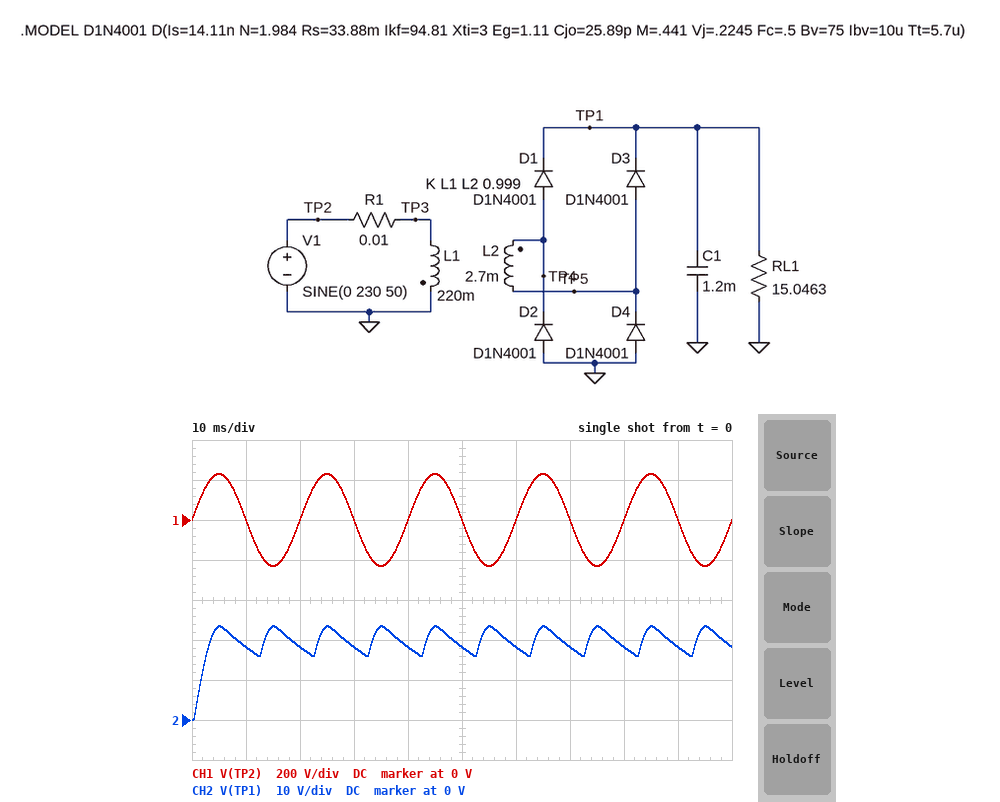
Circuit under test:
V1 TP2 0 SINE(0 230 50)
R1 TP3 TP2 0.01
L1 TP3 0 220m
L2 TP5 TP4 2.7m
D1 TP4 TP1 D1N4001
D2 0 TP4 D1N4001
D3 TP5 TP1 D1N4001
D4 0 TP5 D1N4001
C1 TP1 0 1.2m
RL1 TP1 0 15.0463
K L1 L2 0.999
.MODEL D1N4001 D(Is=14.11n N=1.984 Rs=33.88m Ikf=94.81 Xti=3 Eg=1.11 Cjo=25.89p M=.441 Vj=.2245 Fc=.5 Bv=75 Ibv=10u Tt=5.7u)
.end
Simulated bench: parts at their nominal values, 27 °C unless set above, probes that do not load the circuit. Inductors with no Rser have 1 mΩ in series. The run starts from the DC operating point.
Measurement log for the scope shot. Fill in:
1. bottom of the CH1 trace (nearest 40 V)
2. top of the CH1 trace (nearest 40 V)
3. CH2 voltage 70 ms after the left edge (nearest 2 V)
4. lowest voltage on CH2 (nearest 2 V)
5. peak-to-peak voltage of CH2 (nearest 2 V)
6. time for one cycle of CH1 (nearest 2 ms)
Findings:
-240 V
240 V
18 V
0 V
24 V
20 ms
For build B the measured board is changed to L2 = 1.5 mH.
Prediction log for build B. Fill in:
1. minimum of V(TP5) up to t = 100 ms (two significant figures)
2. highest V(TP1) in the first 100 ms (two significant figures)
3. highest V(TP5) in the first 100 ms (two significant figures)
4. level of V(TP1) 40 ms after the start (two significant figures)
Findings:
-1.2 V
17 V
18 V
13 V
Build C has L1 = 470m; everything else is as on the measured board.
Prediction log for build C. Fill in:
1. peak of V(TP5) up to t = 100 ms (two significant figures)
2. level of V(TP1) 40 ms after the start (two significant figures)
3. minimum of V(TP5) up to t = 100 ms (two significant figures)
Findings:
16 V
12 V
-1.2 V
